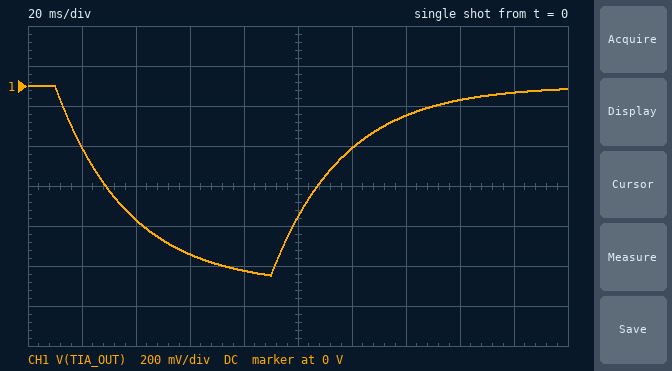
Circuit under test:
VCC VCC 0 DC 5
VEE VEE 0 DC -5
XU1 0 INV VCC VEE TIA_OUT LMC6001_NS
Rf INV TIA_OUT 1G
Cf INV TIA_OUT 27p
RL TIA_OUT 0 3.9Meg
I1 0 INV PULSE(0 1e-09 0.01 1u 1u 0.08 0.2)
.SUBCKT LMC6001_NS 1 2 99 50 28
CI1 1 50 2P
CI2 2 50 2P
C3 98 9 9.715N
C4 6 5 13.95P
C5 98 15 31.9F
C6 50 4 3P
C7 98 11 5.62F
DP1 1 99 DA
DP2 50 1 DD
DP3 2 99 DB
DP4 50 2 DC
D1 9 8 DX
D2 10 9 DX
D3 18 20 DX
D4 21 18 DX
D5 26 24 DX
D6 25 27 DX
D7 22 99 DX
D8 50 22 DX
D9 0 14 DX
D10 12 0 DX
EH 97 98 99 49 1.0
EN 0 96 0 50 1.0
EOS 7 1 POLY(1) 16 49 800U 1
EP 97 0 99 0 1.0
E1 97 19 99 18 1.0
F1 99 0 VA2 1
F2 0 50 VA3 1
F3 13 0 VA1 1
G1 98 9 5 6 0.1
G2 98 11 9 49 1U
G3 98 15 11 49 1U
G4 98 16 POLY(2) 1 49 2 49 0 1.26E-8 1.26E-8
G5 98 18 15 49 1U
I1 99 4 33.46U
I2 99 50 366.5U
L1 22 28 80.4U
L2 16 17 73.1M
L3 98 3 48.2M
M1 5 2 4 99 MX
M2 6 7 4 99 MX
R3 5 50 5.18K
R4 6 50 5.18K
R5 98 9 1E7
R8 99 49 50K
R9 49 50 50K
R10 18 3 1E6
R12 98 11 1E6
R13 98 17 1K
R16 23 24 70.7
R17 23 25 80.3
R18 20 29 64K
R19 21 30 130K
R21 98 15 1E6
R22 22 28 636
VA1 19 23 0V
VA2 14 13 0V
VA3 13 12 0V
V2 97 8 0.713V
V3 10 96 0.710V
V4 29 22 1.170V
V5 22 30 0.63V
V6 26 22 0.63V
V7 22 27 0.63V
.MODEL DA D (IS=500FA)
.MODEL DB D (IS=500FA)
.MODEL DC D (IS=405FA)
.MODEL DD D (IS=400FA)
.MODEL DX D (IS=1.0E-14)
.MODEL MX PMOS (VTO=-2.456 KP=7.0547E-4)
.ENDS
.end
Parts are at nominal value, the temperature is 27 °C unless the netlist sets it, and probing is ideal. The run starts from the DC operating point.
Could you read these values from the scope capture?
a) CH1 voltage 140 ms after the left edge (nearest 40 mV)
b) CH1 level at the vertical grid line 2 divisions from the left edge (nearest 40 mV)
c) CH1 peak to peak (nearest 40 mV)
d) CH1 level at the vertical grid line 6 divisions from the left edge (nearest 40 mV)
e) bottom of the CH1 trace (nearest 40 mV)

-160 mV
-680 mV
960 mV
-320 mV
-960 mV
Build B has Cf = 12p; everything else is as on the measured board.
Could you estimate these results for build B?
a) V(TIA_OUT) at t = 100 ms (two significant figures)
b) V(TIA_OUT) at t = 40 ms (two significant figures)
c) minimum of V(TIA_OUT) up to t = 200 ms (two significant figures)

-430 mV
-920 mV
-1.0 V
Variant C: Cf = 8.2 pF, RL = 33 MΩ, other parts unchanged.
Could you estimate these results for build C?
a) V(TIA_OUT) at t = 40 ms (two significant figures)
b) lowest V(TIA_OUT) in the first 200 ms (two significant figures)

-970 mV
-1.0 V
